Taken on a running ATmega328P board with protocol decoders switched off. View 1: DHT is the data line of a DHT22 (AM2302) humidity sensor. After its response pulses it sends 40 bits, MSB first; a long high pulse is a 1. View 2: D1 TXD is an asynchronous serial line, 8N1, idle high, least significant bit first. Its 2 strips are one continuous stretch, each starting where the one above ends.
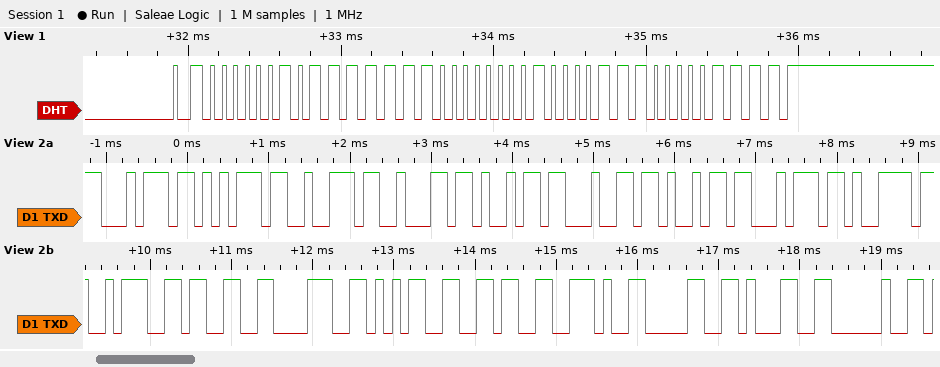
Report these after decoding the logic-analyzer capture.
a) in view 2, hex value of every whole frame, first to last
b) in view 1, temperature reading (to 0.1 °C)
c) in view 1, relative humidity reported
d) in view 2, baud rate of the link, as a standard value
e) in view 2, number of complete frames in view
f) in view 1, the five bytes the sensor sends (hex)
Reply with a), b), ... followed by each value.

a) 74 75 72 62 69 64 69 74 79 3A 33 38 35 36 2E 30 31 20
b) 27.0 °C
c) 76.6 %
d) 9600 baud
e) 18
f) 02 FE 01 0E 0F
